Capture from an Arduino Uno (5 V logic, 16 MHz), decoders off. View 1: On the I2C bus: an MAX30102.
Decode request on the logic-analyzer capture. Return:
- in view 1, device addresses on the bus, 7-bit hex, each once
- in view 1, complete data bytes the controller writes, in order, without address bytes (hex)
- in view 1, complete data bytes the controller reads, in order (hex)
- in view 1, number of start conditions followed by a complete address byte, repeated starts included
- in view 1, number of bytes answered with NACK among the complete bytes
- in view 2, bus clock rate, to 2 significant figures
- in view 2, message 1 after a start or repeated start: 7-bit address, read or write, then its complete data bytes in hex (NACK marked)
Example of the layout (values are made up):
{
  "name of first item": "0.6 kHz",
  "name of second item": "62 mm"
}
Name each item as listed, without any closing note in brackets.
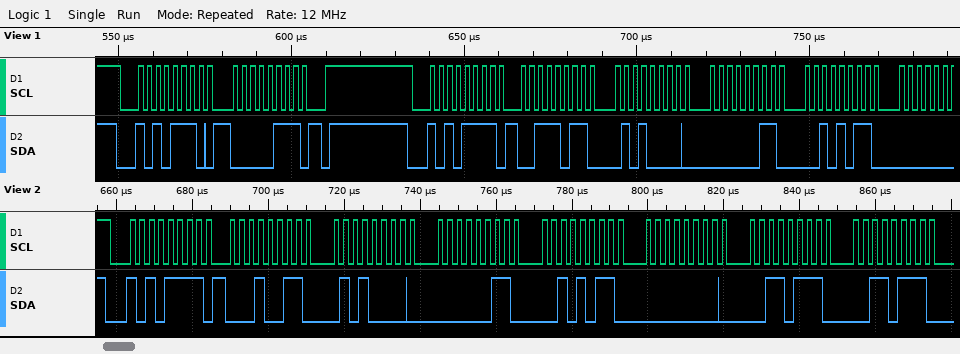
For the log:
{
  "in view 1, device addresses on the bus, 7-bit hex, each once": "0x57",
  "in view 1, complete data bytes the controller writes, in order, without address bytes": "07",
  "in view 1, complete data bytes the controller reads, in order": "3B 50 03 2B",
  "in view 1, number of start conditions followed by a complete address byte, repeated starts included": "2",
  "in view 1, number of bytes answered with NACK among the complete bytes": "0",
  "in view 2, bus clock rate, to 2 significant figures": "400 kHz",
  "in view 2, message 1 after a start or repeated start: 7-bit address, read or write, then its complete data bytes in hex": "0x57 read: 13 50 03 2B 00 37 37"
}
